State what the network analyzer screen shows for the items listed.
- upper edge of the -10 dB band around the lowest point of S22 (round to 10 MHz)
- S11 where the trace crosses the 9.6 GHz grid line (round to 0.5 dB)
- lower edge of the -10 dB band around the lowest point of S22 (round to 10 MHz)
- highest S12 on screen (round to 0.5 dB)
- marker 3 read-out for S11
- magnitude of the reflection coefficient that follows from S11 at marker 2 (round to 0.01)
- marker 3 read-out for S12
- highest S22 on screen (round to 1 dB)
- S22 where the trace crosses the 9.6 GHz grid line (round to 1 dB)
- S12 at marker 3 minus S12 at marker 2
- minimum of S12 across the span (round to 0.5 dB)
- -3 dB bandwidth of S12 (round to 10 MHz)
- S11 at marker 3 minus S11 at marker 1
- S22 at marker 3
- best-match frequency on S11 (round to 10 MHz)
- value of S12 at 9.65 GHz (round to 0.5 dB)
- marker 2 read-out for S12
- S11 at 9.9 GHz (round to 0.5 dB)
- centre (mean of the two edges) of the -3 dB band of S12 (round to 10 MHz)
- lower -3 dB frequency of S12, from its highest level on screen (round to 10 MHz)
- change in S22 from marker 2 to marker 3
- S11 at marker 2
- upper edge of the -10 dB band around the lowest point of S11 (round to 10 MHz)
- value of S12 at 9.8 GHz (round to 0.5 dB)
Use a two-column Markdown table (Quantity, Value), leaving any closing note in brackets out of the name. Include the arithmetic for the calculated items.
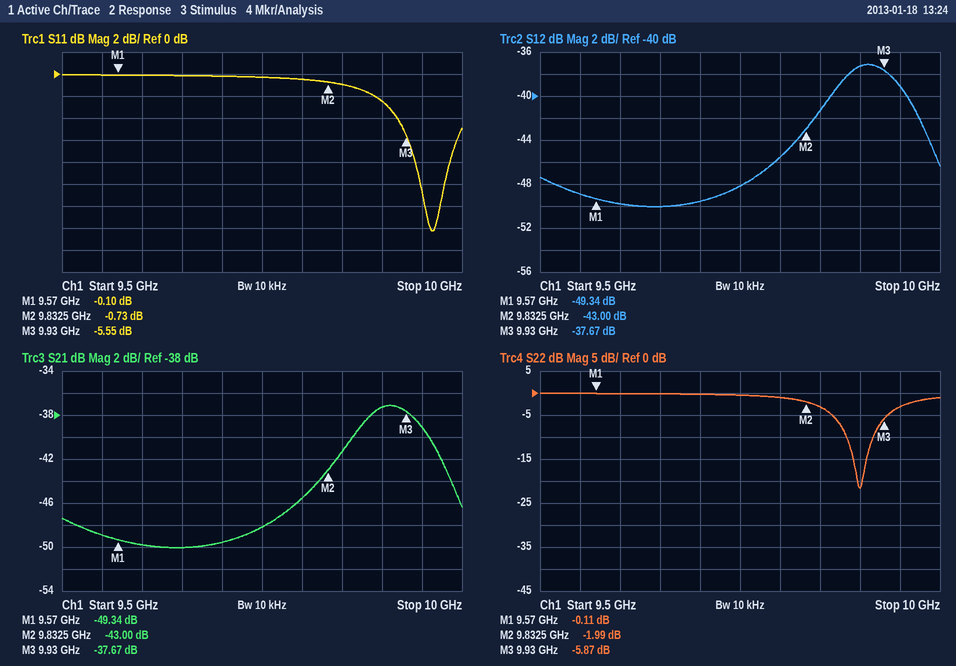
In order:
| Quantity | Value |
|---|---|
| upper edge of the -10 dB band around the lowest point of S22 | 9.92 GHz |
| S11 where the trace crosses the 9.6 GHz grid line | 0.0 dB |
| lower edge of the -10 dB band around the lowest point of S22 | 9.88 GHz |
| highest S12 on screen | -37.0 dB |
| marker 3 read-out for S11 | -5.55 dB |
| magnitude of the reflection coefficient that follows from S11 at marker 2 | 10^(-0.73/20) ≈ 0.92 |
| marker 3 read-out for S12 | -37.67 dB |
| highest S22 on screen | 0 dB |
| S22 where the trace crosses the 9.6 GHz grid line | 0 dB |
| S12 at marker 3 minus S12 at marker 2 | -37.67 − (-43) = 5.33 dB |
| minimum of S12 across the span | -50.0 dB |
| -3 dB bandwidth of S12 | 9.96 GHz − 9.86 GHz = 100 MHz |
| S11 at marker 3 minus S11 at marker 1 | -5.55 − (-0.1) = -5.45 dB |
| S22 at marker 3 | -5.87 dB |
| best-match frequency on S11 | 9.96 GHz |
| value of S12 at 9.65 GHz | -50.0 dB |
| marker 2 read-out for S12 | -43.00 dB |
| S11 at 9.9 GHz | -2.5 dB |
| centre (mean of the two edges) of the -3 dB band of S12 | 9.91 GHz |
| lower -3 dB frequency of S12, from its highest level on screen | 9.86 GHz |
| change in S22 from marker 2 to marker 3 | -5.87 − (-1.99) = -3.88 dB |
| S11 at marker 2 | -0.73 dB |
| upper edge of the -10 dB band around the lowest point of S11 | 9.98 GHz |
| value of S12 at 9.8 GHz | -45.5 dB |
